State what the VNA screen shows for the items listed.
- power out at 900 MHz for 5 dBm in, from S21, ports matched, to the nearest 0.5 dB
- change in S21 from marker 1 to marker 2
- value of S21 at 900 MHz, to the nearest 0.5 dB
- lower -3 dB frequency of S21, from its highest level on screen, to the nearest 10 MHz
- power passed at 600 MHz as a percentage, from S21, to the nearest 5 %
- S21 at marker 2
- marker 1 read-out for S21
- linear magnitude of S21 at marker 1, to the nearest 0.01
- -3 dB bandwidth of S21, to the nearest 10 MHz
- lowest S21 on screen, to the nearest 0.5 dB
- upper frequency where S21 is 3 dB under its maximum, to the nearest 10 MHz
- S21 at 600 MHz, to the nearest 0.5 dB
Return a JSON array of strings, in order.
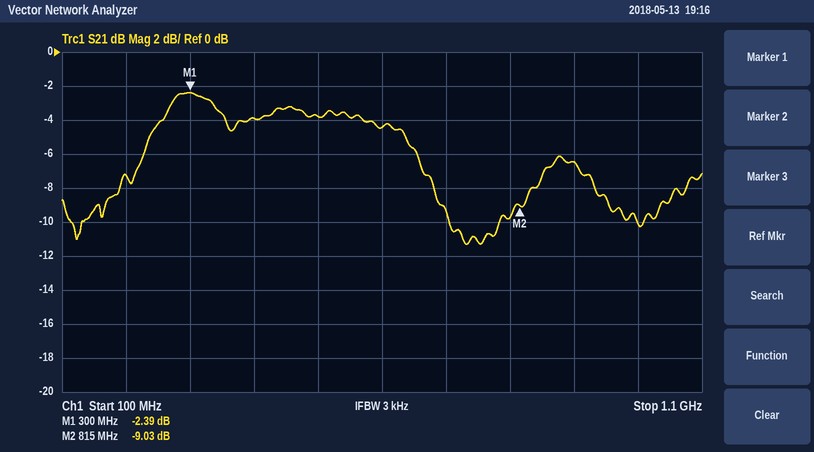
["-1.5 dBm", "-6.64 dB", "-6.5 dB", "230 MHz", "35 %", "-9.03 dB", "-2.39 dB", "0.76", "410 MHz", "-11.5 dB", "640 MHz", "-4.5 dB"]
